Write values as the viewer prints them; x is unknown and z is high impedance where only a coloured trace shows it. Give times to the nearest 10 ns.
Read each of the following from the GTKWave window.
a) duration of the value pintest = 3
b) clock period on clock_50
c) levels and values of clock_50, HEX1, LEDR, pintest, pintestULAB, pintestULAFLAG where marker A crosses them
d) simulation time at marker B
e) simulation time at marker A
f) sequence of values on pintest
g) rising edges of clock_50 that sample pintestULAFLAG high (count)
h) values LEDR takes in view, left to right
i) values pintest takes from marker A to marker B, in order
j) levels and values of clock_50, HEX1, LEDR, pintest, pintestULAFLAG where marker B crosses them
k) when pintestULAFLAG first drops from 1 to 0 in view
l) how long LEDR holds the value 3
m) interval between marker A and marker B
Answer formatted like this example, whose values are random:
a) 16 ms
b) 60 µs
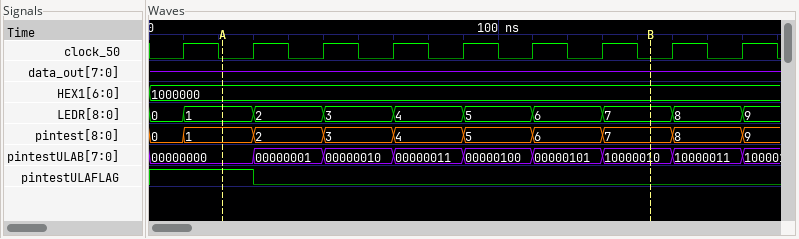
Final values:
a) 20 ns
b) 20 ns
c) clock_50=0, HEX1=1000000, LEDR=1, pintest=1, pintestULAB=00000000, pintestULAFLAG=1
d) 140 ns
e) 20 ns
f) 0, 1, 2, 3, 4, 5, 6, 7, 8, 9
g) 2
h) 0, 1, 2, 3, 4, 5, 6, 7, 8, 9
i) 1, 2, 3, 4, 5, 6, 7
j) clock_50=0, HEX1=1000000, LEDR=7, pintest=7, pintestULAFLAG=0
k) 30 ns
l) 20 ns
m) 120 ns
